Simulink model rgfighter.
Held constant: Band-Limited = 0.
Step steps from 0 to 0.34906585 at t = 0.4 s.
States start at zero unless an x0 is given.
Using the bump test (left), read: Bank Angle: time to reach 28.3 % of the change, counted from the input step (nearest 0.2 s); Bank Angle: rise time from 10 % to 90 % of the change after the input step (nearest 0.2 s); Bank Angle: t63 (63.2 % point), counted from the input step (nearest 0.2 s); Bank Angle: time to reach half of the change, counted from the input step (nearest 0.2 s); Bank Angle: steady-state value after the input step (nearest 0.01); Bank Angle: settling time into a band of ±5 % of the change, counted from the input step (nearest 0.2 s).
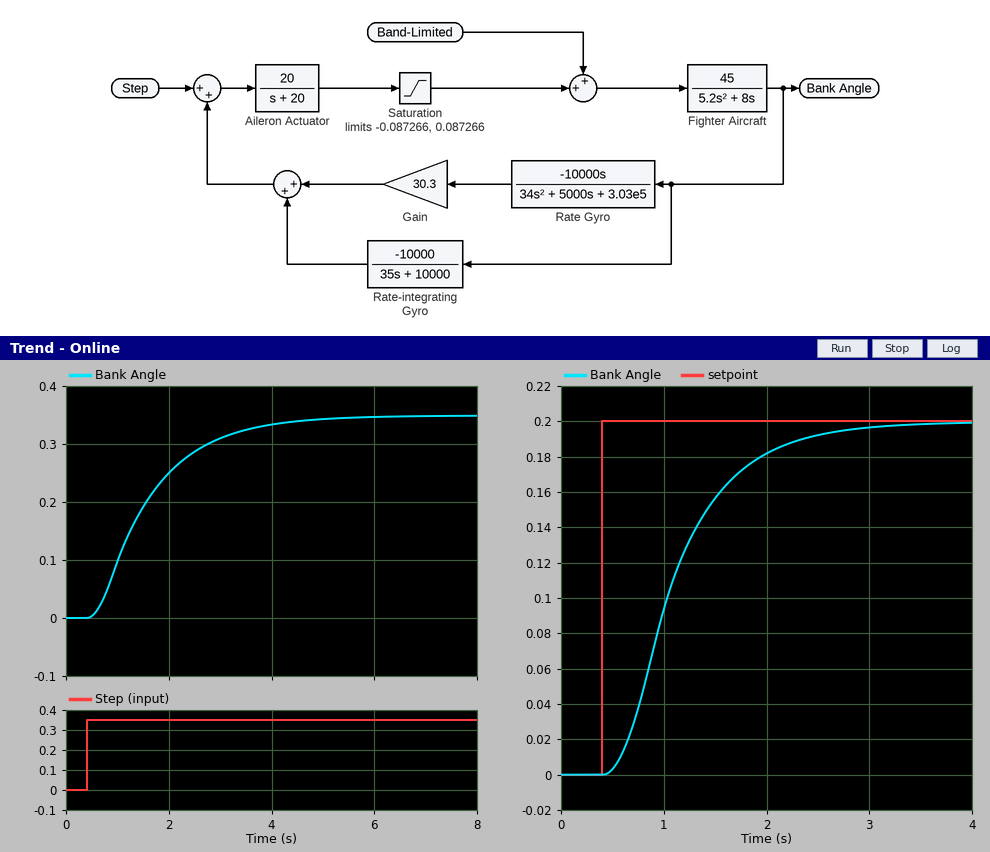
0.6 s
2.4 s
1.4 s
1.0 s
0.35
3.4 s
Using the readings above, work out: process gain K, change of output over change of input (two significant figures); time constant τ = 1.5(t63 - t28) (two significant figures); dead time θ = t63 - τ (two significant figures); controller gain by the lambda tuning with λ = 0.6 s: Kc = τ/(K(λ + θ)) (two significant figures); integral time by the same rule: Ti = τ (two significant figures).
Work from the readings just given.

1.0
1.2 s
0.20 s
1.5
1.2 s
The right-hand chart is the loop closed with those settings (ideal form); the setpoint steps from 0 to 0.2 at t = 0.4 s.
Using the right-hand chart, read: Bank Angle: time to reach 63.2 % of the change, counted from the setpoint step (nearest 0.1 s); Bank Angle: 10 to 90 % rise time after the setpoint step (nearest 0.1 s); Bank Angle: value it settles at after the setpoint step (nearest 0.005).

0.8 s
1.3 s
0.200
